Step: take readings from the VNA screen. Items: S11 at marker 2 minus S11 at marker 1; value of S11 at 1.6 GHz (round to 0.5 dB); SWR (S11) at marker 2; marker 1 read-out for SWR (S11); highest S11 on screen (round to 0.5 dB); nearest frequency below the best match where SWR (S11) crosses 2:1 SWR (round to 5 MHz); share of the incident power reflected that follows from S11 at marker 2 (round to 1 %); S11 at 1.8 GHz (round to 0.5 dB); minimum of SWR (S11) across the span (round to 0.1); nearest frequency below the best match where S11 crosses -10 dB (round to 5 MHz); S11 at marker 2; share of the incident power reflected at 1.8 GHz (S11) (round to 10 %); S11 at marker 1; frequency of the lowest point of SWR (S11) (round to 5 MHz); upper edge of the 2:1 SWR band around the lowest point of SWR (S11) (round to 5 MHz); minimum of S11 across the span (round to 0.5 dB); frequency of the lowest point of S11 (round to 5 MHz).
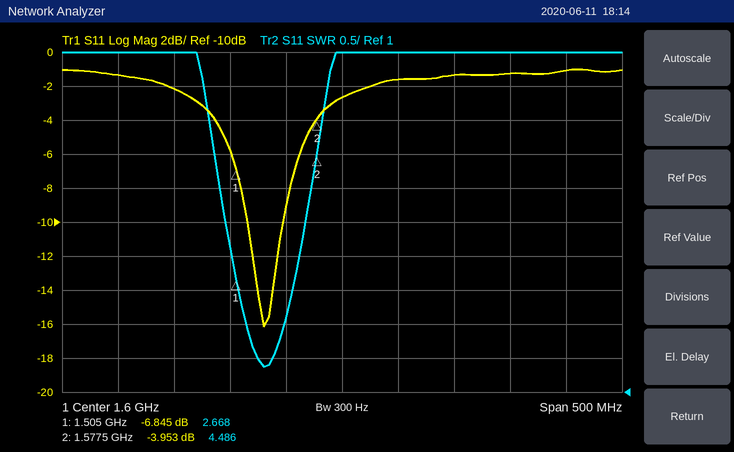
2.892 dB
-2.5 dB
4.486
2.668
-1.0 dB
1.515 GHz
40 %
-1.0 dB
1.4
1.515 GHz
-3.953 dB
80 %
-6.845 dB
1.530 GHz
1.550 GHz
-16.0 dB
1.530 GHz
